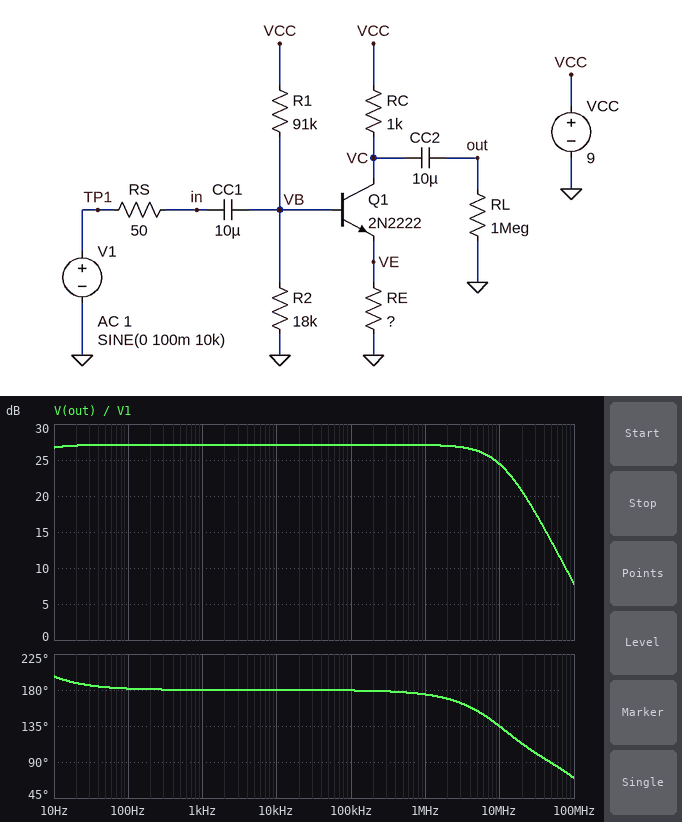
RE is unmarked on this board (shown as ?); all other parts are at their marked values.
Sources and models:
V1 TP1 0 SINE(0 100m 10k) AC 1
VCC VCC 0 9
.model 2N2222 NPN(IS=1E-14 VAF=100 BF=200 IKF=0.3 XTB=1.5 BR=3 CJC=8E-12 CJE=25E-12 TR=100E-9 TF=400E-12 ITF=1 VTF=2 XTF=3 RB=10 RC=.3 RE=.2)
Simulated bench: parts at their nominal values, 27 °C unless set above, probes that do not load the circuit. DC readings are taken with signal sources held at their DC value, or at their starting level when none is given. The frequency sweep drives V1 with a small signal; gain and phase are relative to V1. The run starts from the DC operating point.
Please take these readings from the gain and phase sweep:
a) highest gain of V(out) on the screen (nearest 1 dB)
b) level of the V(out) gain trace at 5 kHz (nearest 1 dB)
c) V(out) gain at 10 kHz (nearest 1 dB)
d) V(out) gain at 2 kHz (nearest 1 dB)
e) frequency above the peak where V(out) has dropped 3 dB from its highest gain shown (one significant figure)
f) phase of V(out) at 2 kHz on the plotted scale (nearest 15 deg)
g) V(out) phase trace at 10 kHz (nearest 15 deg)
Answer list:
27 dB
27 dB
27 dB
27 dB
10 MHz
180 deg
180 deg
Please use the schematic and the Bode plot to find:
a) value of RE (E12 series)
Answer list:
39 Ω
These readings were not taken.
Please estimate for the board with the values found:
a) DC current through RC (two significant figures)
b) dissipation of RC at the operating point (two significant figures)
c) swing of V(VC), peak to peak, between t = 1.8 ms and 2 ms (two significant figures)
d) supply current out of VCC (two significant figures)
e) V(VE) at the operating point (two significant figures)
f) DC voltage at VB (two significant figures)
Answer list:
6.8 mA
46 mW
4.1 V
6.9 mA
270 mV
970 mV
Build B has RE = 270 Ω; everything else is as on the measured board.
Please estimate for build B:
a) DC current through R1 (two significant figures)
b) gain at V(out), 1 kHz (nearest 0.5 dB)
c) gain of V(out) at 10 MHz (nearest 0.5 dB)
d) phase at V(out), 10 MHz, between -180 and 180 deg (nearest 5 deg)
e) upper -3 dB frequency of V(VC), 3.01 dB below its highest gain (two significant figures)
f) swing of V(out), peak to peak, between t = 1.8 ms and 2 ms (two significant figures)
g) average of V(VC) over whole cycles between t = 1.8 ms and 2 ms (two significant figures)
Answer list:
84 µA
11.0 dB
10.5 dB
155 deg
33 MHz
700 mV
6.6 V
